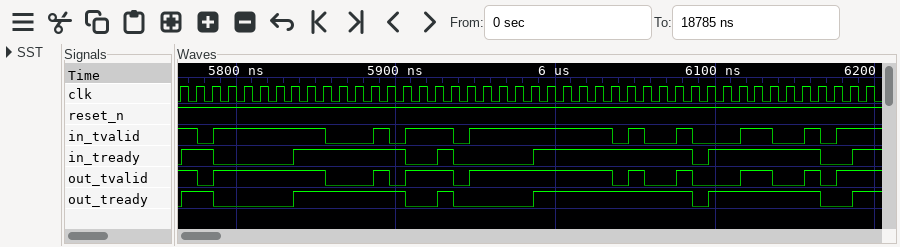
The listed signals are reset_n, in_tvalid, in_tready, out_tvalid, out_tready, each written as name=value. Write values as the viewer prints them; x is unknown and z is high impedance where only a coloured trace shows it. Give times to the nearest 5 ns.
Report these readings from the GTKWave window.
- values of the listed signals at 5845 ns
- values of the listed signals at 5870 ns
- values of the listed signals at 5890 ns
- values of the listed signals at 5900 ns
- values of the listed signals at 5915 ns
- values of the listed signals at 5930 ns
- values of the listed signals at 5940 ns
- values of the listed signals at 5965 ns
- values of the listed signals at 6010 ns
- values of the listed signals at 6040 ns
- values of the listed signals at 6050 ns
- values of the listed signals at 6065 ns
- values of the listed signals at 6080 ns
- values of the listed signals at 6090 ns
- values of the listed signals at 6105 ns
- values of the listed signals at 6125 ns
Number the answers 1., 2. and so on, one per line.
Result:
1. reset_n=1, in_tvalid=1, in_tready=1, out_tvalid=1, out_tready=1
2. reset_n=1, in_tvalid=0, in_tready=1, out_tvalid=0, out_tready=1
3. reset_n=1, in_tvalid=1, in_tready=1, out_tvalid=1, out_tready=1
4. reset_n=1, in_tvalid=0, in_tready=1, out_tvalid=0, out_tready=1
5. reset_n=1, in_tvalid=1, in_tready=0, out_tvalid=1, out_tready=0
6. reset_n=1, in_tvalid=1, in_tready=1, out_tvalid=1, out_tready=1
7. reset_n=1, in_tvalid=0, in_tready=0, out_tvalid=0, out_tready=0
8. reset_n=1, in_tvalid=1, in_tready=0, out_tvalid=1, out_tready=0
9. reset_n=1, in_tvalid=1, in_tready=1, out_tvalid=1, out_tready=1
10. reset_n=1, in_tvalid=0, in_tready=1, out_tvalid=0, out_tready=1
11. reset_n=1, in_tvalid=1, in_tready=1, out_tvalid=1, out_tready=1
12. reset_n=1, in_tvalid=0, in_tready=1, out_tvalid=0, out_tready=1
13. reset_n=1, in_tvalid=1, in_tready=1, out_tvalid=1, out_tready=1
14. reset_n=1, in_tvalid=0, in_tready=0, out_tvalid=0, out_tready=0
15. reset_n=1, in_tvalid=0, in_tready=1, out_tvalid=0, out_tready=1
16. reset_n=1, in_tvalid=1, in_tready=1, out_tvalid=1, out_tready=1
